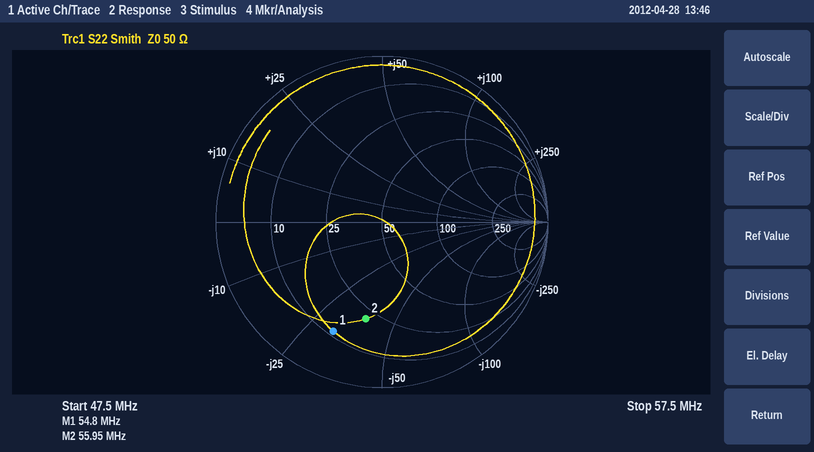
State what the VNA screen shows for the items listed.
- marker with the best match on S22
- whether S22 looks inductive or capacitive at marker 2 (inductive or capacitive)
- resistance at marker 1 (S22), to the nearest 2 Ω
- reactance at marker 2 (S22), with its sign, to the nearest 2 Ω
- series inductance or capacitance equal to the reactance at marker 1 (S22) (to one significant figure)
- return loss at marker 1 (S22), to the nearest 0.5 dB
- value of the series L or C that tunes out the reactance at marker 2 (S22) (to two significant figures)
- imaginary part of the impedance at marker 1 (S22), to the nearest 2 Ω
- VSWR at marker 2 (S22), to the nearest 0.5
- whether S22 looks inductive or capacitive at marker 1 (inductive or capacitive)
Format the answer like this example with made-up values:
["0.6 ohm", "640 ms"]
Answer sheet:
["marker 2", "capacitive", "12 Ω", "-38 Ω", "90 pF", "3.0 dB", "110 nH", "-32 Ω", "4.0", "capacitive"]
